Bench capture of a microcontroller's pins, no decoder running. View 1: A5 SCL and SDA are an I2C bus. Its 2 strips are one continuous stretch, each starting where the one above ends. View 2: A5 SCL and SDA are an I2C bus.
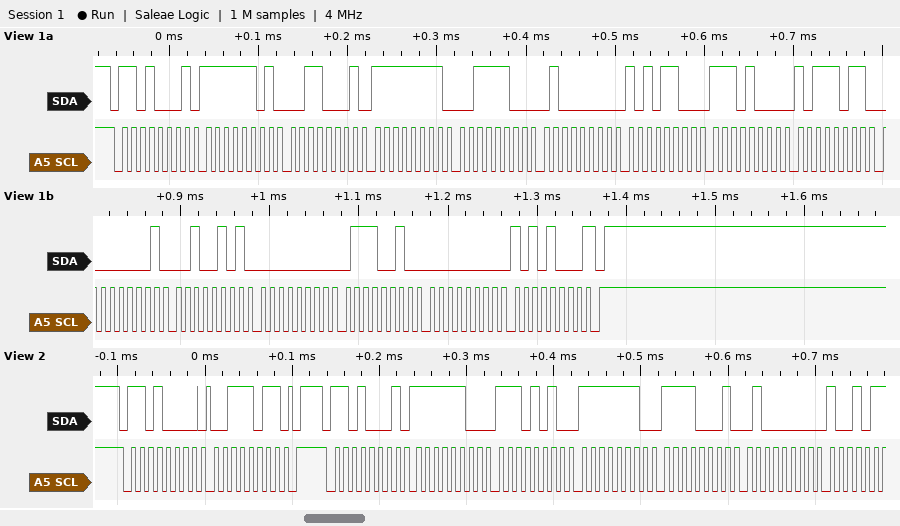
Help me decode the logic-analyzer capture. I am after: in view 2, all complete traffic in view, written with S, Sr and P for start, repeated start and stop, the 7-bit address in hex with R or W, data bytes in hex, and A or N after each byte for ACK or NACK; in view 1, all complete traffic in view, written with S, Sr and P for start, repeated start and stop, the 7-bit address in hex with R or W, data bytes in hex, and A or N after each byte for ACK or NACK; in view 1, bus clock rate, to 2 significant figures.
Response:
S 68W A 3B A P S 68R A FC A EA A FE A F1 A 40 A
S 68R A FD A 31 A FF A 3C A 40 A AC A E8 A BB A 01 A 25 A 00 A 72 A 00 A A8 N P
100 kHz
